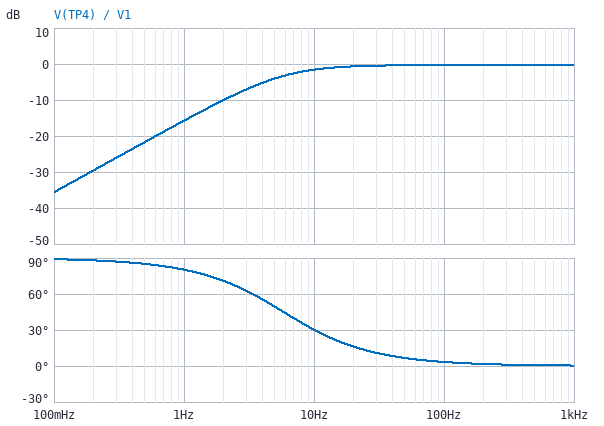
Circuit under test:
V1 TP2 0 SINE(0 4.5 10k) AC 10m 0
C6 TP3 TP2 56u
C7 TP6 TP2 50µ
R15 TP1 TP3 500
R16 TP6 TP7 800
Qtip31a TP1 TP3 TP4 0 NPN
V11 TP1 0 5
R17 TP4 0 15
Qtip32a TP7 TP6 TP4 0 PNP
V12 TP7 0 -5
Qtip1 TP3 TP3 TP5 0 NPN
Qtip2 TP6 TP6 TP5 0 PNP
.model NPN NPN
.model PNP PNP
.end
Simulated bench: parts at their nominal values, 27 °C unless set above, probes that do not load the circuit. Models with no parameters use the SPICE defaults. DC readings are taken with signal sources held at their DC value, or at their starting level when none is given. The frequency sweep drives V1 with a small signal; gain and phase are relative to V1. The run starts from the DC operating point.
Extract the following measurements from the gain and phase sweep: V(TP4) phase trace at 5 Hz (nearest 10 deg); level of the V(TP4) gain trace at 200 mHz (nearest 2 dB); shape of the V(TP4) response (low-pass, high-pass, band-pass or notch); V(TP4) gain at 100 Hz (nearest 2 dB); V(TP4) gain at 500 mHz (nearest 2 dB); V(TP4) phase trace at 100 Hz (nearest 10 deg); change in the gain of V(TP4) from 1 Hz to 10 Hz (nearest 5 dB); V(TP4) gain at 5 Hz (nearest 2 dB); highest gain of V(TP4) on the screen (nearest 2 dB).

50 deg
-30 dB
high-pass
0 dB
-22 dB
0 deg
15 dB
-4 dB
0 dB
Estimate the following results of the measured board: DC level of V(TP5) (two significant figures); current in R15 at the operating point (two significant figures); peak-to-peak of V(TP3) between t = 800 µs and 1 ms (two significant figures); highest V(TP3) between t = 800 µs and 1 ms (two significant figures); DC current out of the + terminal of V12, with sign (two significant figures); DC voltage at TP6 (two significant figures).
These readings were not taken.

810 mV
6.7 mA
9.0 V
5.9 V
-7.0 mA
-11 mV
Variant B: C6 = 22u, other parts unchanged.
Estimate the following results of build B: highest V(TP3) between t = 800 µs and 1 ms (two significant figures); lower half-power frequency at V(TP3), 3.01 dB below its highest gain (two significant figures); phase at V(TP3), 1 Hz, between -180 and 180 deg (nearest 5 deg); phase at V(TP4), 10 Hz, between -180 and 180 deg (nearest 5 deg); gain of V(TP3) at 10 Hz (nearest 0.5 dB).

5.9 V
8.7 Hz
85 deg
40 deg
-2.5 dB
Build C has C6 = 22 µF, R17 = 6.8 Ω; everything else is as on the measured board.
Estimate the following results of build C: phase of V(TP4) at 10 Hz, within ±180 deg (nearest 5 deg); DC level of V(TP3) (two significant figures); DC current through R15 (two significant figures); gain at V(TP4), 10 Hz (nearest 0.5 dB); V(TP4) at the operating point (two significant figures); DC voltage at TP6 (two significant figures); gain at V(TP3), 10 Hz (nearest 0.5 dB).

45 deg
1.5 V
7.0 mA
-3.5 dB
620 mV
-130 mV
-3.0 dB
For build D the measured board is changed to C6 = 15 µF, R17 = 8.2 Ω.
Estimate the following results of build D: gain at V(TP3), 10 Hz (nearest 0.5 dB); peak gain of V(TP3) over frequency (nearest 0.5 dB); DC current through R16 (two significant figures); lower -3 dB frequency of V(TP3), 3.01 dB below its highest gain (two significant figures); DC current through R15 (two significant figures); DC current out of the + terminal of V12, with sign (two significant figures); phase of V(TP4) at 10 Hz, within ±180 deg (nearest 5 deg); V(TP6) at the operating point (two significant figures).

-3.5 dB
0 dB
6.1 mA
11 Hz
6.9 mA
-6.6 mA
45 deg
-100 mV
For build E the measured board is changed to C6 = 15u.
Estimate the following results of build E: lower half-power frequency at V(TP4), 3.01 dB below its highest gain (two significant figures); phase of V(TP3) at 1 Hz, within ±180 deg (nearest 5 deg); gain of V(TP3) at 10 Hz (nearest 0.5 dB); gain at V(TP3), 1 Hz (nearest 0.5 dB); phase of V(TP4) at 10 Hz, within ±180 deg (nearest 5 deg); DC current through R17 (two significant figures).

9.7 Hz
85 deg
-3.0 dB
-19.5 dB
45 deg
50 mA
